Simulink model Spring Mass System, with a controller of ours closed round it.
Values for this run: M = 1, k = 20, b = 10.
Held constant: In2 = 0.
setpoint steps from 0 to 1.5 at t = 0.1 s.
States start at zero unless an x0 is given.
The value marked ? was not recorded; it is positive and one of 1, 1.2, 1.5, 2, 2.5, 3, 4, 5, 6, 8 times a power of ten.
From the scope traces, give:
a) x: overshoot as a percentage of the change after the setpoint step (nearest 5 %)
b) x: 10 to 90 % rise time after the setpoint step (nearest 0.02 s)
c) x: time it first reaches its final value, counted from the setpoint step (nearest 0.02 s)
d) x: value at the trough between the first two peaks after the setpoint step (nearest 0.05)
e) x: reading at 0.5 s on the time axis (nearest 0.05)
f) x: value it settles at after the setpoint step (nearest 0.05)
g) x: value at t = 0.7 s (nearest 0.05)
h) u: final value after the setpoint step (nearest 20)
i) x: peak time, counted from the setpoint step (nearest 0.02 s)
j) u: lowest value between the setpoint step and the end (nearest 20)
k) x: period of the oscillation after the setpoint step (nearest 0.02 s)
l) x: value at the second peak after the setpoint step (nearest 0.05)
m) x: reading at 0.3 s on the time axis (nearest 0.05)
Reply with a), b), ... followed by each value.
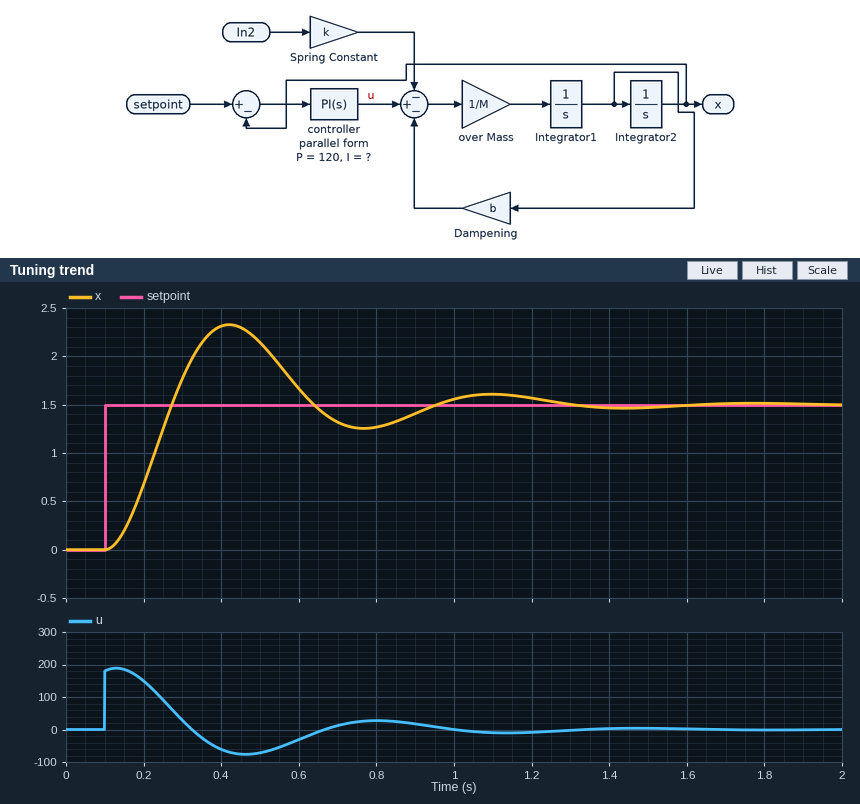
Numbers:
a) 55 %
b) 0.12 s
c) 0.18 s
d) 1.25
e) 2.15
f) 1.50
g) 1.30
h) 0
i) 0.32 s
j) -80
k) 0.68 s
l) 1.60
m) 1.75
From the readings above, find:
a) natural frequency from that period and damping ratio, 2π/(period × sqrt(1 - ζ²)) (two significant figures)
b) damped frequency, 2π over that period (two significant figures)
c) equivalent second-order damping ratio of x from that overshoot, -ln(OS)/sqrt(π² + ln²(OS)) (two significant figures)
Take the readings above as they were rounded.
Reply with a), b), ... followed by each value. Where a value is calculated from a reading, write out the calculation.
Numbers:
a) 2π / (0.68 × sqrt(1 - 0.19²)) = 9.4 rad/s
b) 2π / 0.68 = 9.2 rad/s
c) ln(0.55) = -0.598; 0.598 / sqrt(9.870 + 0.357) = 0.19
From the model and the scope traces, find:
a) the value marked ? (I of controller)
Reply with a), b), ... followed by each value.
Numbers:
a) 400
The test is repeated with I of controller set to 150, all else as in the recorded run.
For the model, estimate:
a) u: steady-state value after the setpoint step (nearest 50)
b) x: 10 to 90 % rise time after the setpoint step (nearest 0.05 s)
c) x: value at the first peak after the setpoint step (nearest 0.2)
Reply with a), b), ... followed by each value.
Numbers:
a) 0
b) 0.15 s
c) 2.0
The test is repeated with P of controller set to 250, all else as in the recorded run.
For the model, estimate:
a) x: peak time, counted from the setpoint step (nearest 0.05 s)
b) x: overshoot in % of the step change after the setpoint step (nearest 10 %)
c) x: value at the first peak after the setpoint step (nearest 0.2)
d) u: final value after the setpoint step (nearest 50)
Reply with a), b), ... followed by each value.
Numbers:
a) 0.20 s
b) 50 %
c) 2.2
d) 0
